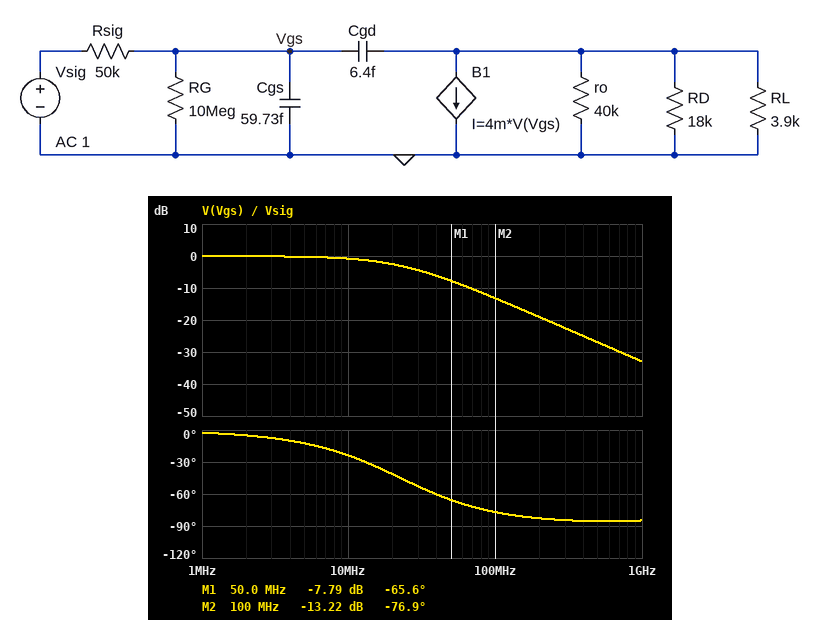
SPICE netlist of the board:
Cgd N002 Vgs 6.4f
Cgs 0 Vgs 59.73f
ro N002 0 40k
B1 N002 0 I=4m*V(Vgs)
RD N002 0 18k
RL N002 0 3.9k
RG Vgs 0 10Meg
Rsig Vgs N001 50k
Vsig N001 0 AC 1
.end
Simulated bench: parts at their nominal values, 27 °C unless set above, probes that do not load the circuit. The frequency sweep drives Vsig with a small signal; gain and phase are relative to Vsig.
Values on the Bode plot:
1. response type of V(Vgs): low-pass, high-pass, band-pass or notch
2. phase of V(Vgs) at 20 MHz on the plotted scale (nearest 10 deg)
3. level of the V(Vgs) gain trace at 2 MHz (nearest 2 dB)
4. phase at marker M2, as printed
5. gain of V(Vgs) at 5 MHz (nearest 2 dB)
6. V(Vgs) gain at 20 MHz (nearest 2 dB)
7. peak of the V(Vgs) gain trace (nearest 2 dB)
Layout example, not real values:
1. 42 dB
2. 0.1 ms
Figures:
1. low-pass
2. -40 deg
3. 0 dB
4. -76.9 deg
5. 0 dB
6. -2 dB
7. 0 dB
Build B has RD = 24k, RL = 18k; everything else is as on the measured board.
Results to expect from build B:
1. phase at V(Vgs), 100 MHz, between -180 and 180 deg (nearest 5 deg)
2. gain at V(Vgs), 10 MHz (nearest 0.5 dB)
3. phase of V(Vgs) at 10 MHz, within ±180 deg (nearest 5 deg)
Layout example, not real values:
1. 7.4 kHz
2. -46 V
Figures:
1. -80 deg
2. -2.5 dB
3. -40 deg
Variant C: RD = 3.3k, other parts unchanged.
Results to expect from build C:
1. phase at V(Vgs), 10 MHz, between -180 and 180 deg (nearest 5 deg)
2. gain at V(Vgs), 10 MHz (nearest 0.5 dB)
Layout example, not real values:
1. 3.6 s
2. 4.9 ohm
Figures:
1. -20 deg
2. -0.5 dB
